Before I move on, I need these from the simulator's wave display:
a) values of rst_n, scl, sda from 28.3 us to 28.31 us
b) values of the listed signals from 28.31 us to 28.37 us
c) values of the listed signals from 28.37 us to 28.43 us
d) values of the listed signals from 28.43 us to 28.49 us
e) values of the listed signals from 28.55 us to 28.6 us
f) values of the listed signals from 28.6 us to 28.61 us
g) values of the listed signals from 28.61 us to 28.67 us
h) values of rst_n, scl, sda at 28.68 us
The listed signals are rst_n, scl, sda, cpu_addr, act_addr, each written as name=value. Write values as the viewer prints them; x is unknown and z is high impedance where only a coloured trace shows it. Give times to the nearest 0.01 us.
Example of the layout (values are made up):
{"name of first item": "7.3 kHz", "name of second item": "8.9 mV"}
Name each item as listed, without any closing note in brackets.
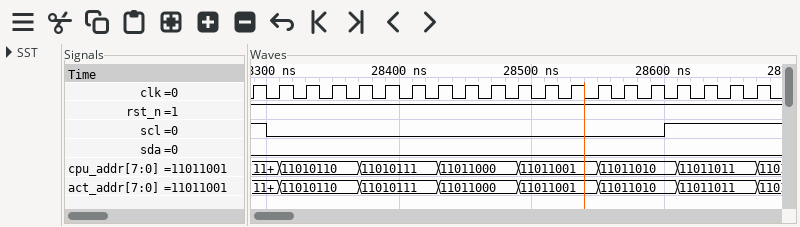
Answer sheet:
{"values of rst_n, scl, sda from 28.3 us to 28.31 us": "rst_n=1, scl=0, sda=0", "values of the listed signals from 28.31 us to 28.37 us": "rst_n=1, scl=0, sda=0, cpu_addr=11010110, act_addr=11010110", "values of the listed signals from 28.37 us to 28.43 us": "rst_n=1, scl=0, sda=0, cpu_addr=11010111, act_addr=11010111", "values of the listed signals from 28.43 us to 28.49 us": "rst_n=1, scl=0, sda=0, cpu_addr=11011000, act_addr=11011000", "values of the listed signals from 28.55 us to 28.6 us": "rst_n=1, scl=0, sda=0, cpu_addr=11011010, act_addr=11011010", "values of the listed signals from 28.6 us to 28.61 us": "rst_n=1, scl=1, sda=0, cpu_addr=11011010, act_addr=11011010", "values of the listed signals from 28.61 us to 28.67 us": "rst_n=1, scl=1, sda=0, cpu_addr=11011011, act_addr=11011011", "values of rst_n, scl, sda at 28.68 us": "rst_n=1, scl=1, sda=0"}
